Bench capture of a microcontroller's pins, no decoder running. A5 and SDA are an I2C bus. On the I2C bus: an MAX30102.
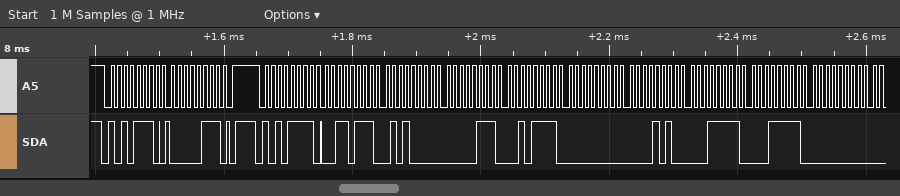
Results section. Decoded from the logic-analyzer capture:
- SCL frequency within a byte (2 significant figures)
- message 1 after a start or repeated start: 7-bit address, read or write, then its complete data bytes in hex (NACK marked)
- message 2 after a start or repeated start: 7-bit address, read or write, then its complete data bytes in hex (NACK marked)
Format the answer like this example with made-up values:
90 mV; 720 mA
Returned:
100 kHz; 0x57 write: 07; 0x57 read: 37 50 07 2F 00 0A 1F 1F 00
